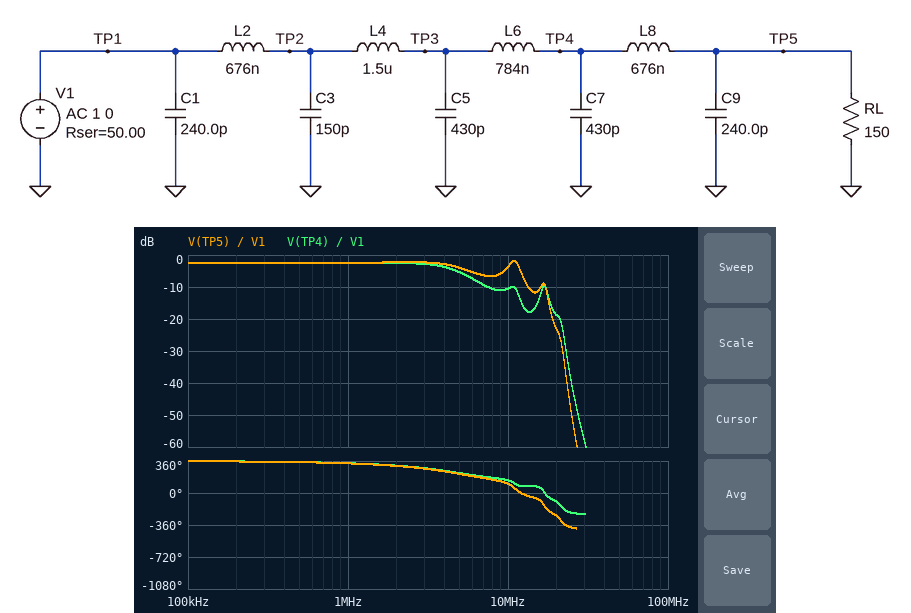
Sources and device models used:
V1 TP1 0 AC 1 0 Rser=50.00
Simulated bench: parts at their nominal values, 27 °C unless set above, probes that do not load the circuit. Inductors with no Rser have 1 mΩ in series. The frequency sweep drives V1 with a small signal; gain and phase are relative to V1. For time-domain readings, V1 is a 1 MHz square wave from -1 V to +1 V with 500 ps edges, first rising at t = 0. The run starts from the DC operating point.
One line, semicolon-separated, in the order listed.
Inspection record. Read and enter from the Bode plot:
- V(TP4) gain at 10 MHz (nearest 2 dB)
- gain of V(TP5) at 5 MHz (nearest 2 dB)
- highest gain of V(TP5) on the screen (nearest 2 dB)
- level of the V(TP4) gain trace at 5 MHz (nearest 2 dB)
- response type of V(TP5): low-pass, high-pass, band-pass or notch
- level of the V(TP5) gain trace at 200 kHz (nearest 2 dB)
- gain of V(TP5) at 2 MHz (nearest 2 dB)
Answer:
-10 dB; -4 dB; -2 dB; -6 dB; low-pass; -2 dB; -2 dB
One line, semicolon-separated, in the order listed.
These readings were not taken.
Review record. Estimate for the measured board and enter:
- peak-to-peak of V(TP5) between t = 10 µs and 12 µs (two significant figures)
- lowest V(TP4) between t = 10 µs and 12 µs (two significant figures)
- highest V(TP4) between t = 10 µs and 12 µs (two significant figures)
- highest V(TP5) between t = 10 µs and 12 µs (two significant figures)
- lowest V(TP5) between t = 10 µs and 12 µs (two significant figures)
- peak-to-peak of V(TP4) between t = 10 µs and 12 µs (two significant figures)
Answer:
1.8 V; -870 mV; 870 mV; 900 mV; -900 mV; 1.7 V
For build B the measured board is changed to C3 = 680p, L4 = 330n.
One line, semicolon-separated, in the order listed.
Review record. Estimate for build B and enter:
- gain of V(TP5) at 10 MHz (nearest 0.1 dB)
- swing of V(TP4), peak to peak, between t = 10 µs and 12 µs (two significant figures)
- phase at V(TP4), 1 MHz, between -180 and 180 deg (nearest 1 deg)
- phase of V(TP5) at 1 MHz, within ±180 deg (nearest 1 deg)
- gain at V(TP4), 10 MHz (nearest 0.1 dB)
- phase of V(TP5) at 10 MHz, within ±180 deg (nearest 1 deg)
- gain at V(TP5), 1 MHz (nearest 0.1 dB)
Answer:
-4.9 dB; 1.6 V; -29 deg; -31 deg; -11.7 dB; 77 deg; -3.0 dB
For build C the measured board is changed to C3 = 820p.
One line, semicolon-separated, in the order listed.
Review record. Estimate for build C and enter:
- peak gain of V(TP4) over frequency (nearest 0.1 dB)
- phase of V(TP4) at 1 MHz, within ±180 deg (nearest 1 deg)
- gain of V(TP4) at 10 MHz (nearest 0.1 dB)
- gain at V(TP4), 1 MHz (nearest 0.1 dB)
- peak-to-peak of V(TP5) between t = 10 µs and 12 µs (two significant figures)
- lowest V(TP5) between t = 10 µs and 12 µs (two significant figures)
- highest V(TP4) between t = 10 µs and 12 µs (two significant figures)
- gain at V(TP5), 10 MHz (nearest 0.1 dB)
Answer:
-2.5 dB; -33 deg; -13.9 dB; -2.9 dB; 1.6 V; -810 mV; 790 mV; -7.1 dB
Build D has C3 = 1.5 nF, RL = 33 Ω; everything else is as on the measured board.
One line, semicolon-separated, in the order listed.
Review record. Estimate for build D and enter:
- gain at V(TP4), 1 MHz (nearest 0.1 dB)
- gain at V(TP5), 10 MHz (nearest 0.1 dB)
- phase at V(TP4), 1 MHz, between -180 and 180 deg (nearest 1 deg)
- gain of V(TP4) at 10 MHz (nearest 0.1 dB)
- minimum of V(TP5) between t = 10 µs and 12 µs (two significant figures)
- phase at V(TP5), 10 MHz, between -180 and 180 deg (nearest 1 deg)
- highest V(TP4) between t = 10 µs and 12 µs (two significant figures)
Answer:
-7.9 dB; -17.8 dB; -29 deg; -15.3 dB; -440 mV; -18 deg; 450 mV
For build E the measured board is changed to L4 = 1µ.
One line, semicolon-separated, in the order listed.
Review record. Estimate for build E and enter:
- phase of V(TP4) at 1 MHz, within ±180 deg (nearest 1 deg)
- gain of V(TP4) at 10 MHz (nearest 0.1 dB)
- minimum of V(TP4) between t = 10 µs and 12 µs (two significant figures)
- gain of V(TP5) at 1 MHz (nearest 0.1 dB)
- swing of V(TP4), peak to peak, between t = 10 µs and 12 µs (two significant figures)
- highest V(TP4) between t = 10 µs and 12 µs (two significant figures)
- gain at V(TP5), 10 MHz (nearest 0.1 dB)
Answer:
-24 deg; -9.8 dB; -800 mV; -2.5 dB; 1.6 V; 800 mV; -3.0 dB
